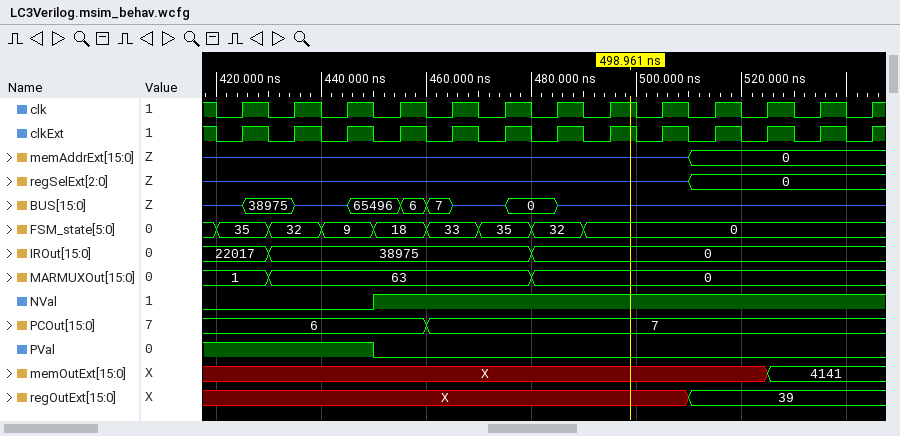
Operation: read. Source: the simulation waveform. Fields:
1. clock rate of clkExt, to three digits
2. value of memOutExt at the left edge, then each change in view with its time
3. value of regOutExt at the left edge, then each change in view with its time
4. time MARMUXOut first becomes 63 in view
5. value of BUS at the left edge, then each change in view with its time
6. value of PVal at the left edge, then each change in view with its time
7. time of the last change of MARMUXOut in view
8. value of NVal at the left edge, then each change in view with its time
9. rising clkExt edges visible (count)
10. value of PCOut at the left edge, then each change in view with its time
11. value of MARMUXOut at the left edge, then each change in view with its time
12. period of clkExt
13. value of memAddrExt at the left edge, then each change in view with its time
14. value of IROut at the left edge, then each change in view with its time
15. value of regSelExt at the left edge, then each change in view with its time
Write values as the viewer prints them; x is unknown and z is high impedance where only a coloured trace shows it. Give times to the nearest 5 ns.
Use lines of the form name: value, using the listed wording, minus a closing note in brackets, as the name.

clock rate of clkExt, to three digits: 100 MHz
value of memOutExt at the left edge, then each change in view with its time: X, 4141 at 525 ns
value of regOutExt at the left edge, then each change in view with its time: X, 39 at 510 ns
time MARMUXOut first becomes 63 in view: 430 ns
value of BUS at the left edge, then each change in view with its time: z, 38975 at 425 ns, z at 435 ns, 65496 at 445 ns, 6 at 455 ns, 7 at 460 ns, z at 465 ns, 0 at 475 ns, z at 485 ns
value of PVal at the left edge, then each change in view with its time: 1, 0 at 450 ns
time of the last change of MARMUXOut in view: 480 ns
value of NVal at the left edge, then each change in view with its time: 0, 1 at 450 ns
rising clkExt edges visible: 13
value of PCOut at the left edge, then each change in view with its time: 6, 7 at 460 ns
value of MARMUXOut at the left edge, then each change in view with its time: 1, 63 at 430 ns, 0 at 480 ns
period of clkExt: 10 ns
value of memAddrExt at the left edge, then each change in view with its time: z, 0 at 510 ns
value of IROut at the left edge, then each change in view with its time: 22017, 38975 at 430 ns, 0 at 480 ns
value of regSelExt at the left edge, then each change in view with its time: z, 0 at 510 ns
